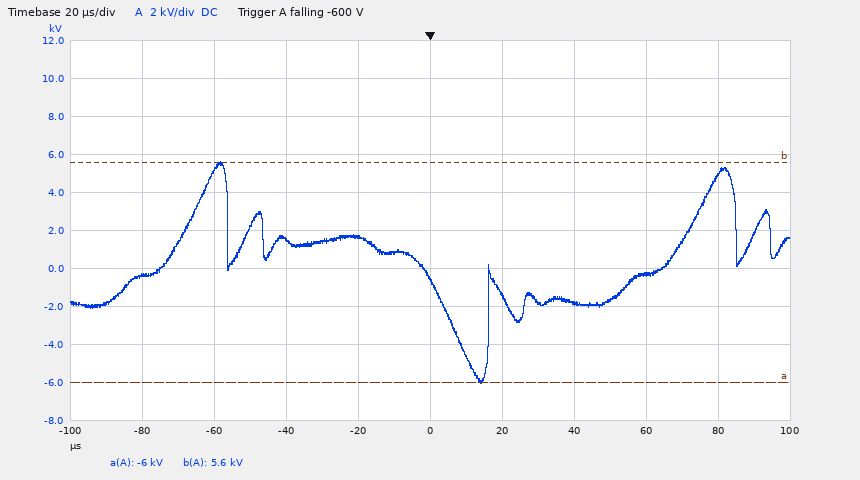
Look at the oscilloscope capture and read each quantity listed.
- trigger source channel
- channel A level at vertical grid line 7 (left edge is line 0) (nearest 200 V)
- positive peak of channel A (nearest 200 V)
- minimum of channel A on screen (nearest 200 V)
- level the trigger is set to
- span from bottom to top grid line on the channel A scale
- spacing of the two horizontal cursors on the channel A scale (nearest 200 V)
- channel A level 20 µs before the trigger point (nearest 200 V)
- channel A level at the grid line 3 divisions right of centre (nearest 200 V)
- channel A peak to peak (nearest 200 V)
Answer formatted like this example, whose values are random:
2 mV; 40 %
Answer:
channel A; -1.8 kV; 5.6 kV; -6.0 kV; -600 V; 20 kV; 11.6 kV; 1.6 kV; -400 V; 11.6 kV
